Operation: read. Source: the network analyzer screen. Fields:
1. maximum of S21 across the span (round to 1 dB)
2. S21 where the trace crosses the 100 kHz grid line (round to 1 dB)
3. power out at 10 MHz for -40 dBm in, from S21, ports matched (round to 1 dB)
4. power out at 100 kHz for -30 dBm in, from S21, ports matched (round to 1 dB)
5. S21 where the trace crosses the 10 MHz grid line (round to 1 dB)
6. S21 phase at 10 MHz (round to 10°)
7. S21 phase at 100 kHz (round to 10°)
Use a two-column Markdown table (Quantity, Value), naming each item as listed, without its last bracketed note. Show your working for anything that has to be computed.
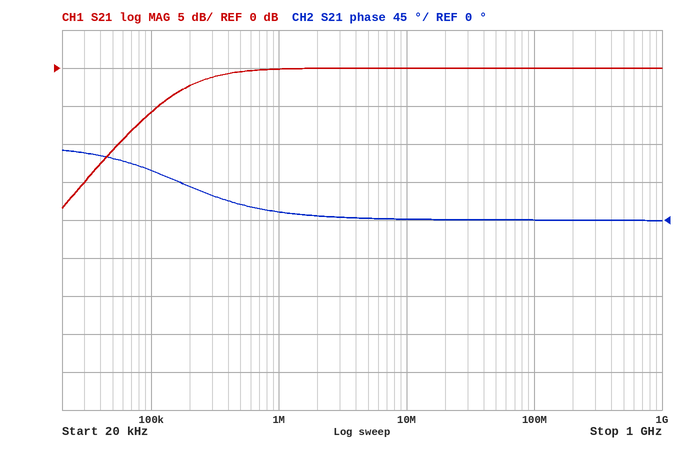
| Quantity | Value |
|---|---|
| maximum of S21 across the span | 0 dB |
| S21 where the trace crosses the 100 kHz grid line | -6 dB |
| power out at 10 MHz for -40 dBm in, from S21, ports matched | -40 dBm + (0 dB) = -40 dBm |
| power out at 100 kHz for -30 dBm in, from S21, ports matched | -30 dBm + (-6 dB) = -36 dBm |
| S21 where the trace crosses the 10 MHz grid line | 0 dB |
| S21 phase at 10 MHz | 0° |
| S21 phase at 100 kHz | 60° |
